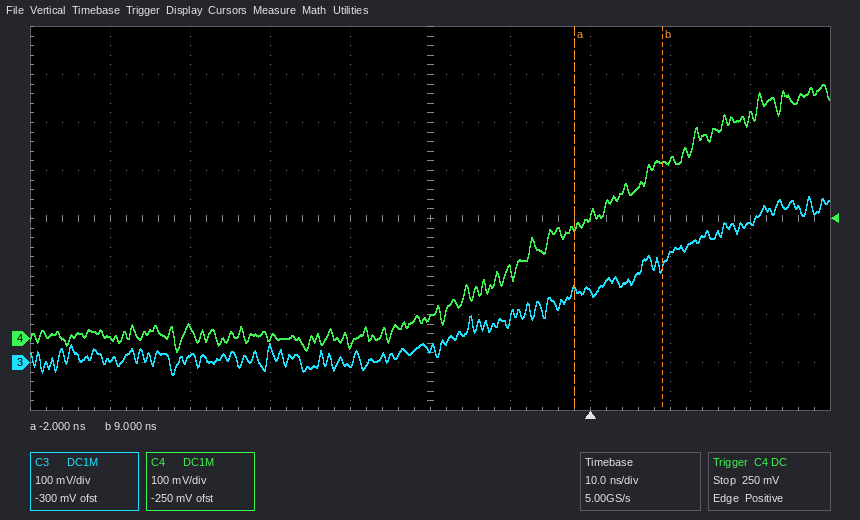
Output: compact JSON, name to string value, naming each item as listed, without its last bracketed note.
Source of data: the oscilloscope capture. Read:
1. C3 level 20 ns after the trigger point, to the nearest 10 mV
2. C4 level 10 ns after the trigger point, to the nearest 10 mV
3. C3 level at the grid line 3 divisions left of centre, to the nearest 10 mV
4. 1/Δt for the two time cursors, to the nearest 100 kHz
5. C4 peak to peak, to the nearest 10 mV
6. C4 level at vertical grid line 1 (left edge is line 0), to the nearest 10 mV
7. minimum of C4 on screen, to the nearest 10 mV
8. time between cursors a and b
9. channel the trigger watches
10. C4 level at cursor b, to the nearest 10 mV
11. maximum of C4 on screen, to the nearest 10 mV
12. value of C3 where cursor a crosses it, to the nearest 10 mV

{"C3 level 20 ns after the trigger point, to the nearest 10 mV": "290 mV", "C4 level 10 ns after the trigger point, to the nearest 10 mV": "370 mV", "C3 level at the grid line 3 divisions left of centre, to the nearest 10 mV": "10 mV", "1/Δt for the two time cursors, to the nearest 100 kHz": "90.9 MHz", "C4 peak to peak, to the nearest 10 mV": "560 mV", "C4 level at vertical grid line 1 (left edge is line 0), to the nearest 10 mV": "0 mV", "minimum of C4 on screen, to the nearest 10 mV": "-30 mV", "time between cursors a and b": "11 ns", "channel the trigger watches": "C4", "C4 level at cursor b, to the nearest 10 mV": "370 mV", "maximum of C4 on screen, to the nearest 10 mV": "530 mV", "value of C3 where cursor a crosses it, to the nearest 10 mV": "150 mV"}
